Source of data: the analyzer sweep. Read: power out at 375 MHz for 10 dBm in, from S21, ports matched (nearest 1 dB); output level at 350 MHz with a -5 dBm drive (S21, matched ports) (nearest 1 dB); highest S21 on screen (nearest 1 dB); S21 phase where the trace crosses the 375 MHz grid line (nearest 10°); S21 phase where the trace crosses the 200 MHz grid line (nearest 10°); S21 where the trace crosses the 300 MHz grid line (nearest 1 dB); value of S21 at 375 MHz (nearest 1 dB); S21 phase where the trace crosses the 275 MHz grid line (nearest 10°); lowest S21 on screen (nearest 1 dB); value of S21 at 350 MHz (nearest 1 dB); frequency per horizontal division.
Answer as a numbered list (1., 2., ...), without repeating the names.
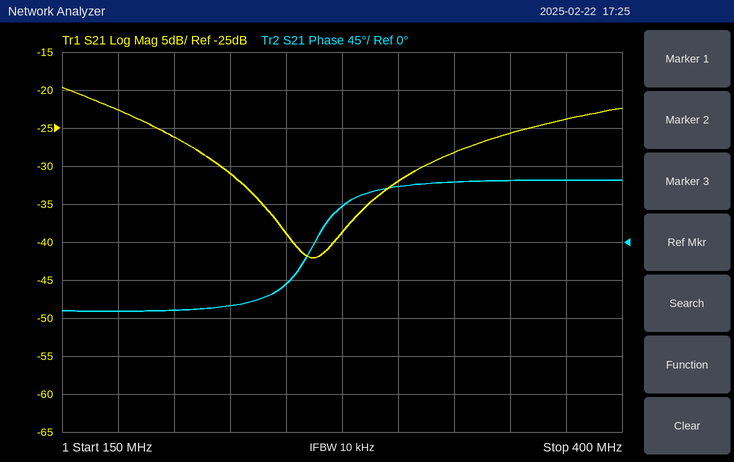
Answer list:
1. -14 dBm
2. -31 dBm
3. -20 dB
4. 70°
5. -80°
6. -32 dB
7. -24 dB
8. 40°
9. -42 dB
10. -26 dB
11. 25 MHz
